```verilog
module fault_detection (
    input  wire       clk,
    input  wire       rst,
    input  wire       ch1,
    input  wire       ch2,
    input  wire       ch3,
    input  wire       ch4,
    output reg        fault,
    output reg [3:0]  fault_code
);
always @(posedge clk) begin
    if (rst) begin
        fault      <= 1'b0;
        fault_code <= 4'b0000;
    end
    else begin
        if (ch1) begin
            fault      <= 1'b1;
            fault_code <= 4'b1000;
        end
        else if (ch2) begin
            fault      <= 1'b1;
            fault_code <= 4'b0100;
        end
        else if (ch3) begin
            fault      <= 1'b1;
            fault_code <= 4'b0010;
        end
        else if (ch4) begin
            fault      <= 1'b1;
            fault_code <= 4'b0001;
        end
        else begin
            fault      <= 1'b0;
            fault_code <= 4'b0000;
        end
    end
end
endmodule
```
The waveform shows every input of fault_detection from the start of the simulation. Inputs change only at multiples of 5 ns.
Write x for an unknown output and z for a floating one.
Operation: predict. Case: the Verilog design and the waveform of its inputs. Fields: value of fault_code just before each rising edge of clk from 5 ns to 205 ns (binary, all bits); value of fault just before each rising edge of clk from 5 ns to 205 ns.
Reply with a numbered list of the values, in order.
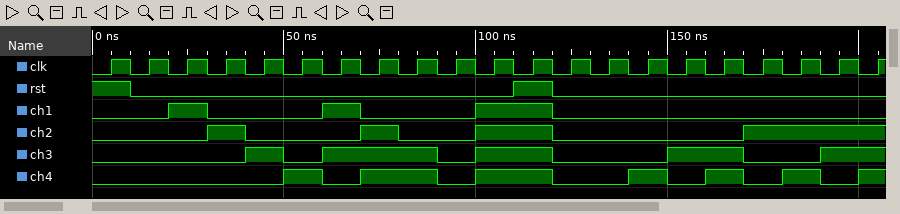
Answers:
1. x, 0000, 0000, 1000, 0100, 0010, 0001, 1000, 0100, 0010, 0000, 1000, 0000, 0000, 0000, 0001, 0010, 0010, 0100, 0100, 0100
2. x 0 0 1 1 1 1 1 1 1 0 1 0 0 0 1 1 1 1 1 1
